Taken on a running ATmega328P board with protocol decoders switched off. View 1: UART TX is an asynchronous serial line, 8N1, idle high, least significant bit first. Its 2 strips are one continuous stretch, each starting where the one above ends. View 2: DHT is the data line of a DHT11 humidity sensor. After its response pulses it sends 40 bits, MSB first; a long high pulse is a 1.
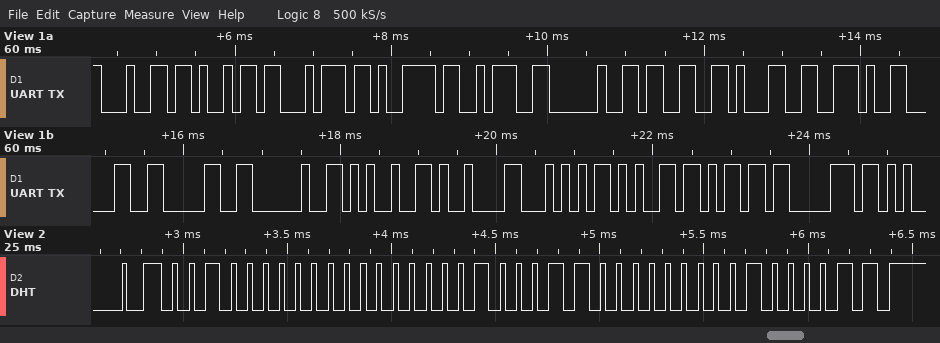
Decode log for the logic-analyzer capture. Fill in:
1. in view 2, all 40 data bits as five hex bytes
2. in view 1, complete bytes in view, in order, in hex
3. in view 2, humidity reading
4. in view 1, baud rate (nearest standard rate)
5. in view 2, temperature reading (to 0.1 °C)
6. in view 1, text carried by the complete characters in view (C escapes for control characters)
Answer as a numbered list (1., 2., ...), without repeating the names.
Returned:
1. 20 00 23 00 43
2. 0x64 0x69 0x74 0x79 0x3A 0x20 0x33 0x31 0x2E 0x30 0x30 0x20 0x25 0x09 0x54 0x65 0x6D 0x70
3. 32 %
4. 9600 baud
5. 35.0 °C
6. "dity: 31.00 %\tTemp"
